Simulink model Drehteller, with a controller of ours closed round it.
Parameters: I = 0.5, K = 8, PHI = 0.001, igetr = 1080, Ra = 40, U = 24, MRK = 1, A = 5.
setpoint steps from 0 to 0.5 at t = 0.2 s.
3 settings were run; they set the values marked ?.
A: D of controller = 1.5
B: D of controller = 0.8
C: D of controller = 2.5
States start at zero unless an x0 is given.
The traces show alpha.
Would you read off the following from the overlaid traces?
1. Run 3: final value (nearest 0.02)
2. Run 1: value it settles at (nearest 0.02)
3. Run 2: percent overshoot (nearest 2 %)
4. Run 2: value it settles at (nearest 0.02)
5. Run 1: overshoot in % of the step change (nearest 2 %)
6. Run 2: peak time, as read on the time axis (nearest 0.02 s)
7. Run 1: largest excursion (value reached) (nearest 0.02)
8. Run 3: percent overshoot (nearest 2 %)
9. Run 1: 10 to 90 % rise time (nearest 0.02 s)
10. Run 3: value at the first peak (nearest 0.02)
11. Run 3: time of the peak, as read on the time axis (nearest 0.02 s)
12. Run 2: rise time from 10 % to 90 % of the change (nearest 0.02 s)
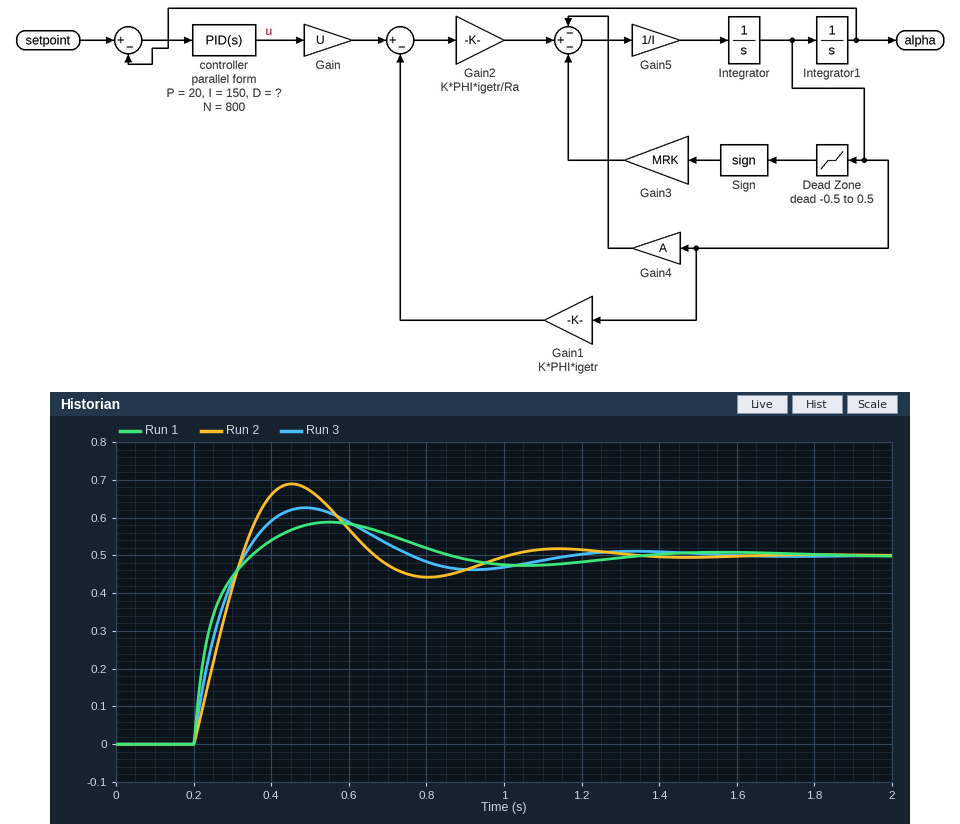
0.50
0.50
38 %
0.50
18 %
0.46 s
0.58
26 %
0.10 s
0.62
0.48 s
0.10 s
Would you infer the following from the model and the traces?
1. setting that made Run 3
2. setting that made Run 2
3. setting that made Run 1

A
B
C
